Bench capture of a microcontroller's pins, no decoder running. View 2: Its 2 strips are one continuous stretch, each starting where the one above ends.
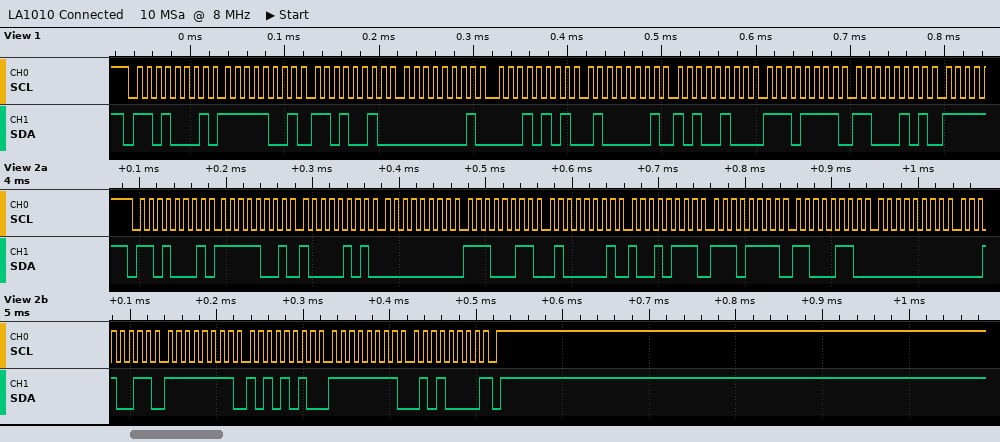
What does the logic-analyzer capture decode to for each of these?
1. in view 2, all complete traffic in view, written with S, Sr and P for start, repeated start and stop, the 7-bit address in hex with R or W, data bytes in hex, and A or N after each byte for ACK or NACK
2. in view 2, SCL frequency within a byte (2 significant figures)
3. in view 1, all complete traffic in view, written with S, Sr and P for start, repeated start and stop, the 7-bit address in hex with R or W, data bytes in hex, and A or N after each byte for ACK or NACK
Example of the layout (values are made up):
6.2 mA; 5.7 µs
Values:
S 68R A F9 A 85 A 00 A E3 A 41 A 97 A EF A C6 A 00 A 13 A FF A AA A FF A 50 N P; 100 kHz; S 68R A F9 A D2 A 01 A 15 A 41 A A4 A EF A C5 A
